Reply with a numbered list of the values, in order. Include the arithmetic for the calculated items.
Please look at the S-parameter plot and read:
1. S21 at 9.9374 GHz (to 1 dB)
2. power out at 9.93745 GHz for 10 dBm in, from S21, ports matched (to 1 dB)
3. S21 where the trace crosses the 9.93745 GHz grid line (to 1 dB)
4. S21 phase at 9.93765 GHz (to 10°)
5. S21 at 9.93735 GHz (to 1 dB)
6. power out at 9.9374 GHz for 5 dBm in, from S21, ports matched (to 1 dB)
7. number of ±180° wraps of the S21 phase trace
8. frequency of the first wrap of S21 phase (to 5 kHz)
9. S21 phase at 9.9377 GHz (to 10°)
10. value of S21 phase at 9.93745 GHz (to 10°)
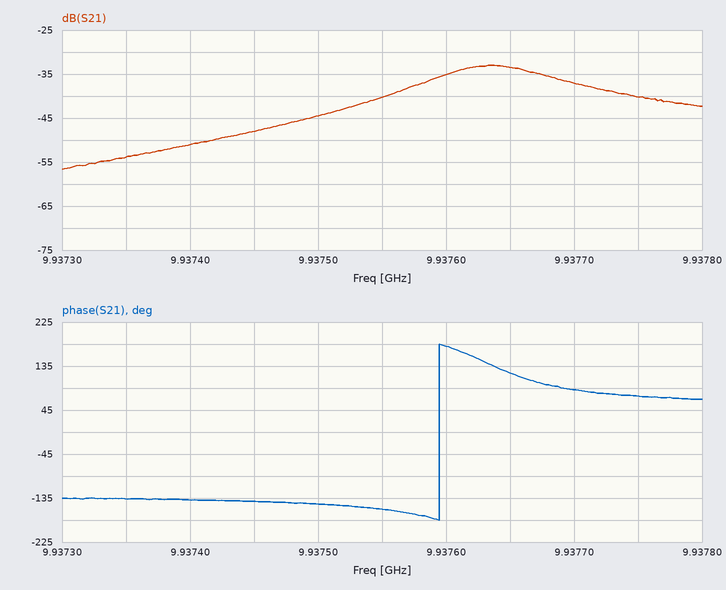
1. -51 dB
2. 10 dBm + (-48 dB) = -38 dBm
3. -48 dB
4. 120°
5. -54 dB
6. 5 dBm + (-51 dB) = -46 dBm
7. 1
8. 9.937595 GHz
9. 90°
10. -140°
